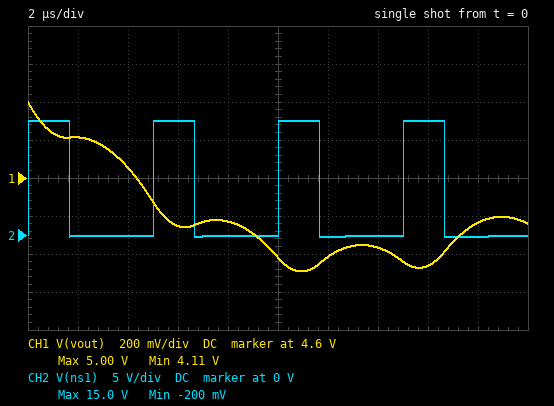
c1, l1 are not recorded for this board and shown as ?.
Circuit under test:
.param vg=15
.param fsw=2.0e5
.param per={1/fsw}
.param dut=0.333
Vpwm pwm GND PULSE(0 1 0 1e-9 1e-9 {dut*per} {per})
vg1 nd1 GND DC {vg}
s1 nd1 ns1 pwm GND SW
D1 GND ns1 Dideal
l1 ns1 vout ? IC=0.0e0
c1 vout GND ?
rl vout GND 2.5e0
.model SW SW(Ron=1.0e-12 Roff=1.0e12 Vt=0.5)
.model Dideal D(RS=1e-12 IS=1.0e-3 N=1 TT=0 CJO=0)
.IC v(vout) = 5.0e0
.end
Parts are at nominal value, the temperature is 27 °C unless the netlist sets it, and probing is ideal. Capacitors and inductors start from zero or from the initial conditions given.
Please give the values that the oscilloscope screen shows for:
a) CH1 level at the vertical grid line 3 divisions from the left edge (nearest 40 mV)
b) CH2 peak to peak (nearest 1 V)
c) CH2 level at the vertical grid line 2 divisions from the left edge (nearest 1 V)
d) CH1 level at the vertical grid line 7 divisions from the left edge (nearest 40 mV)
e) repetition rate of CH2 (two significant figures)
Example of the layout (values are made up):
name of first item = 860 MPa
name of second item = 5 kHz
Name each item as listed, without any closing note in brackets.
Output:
CH1 level at the vertical grid line 3 divisions from the left edge = 4.36 V
CH2 peak to peak = 15 V
CH2 level at the vertical grid line 2 divisions from the left edge = 0 V
CH1 level at the vertical grid line 7 divisions from the left edge = 4.24 V
repetition rate of CH2 = 200 kHz
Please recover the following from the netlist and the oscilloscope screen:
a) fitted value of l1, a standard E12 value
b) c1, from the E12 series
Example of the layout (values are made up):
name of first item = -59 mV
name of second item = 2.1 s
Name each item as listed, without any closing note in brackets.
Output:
fitted value of l1, a standard E12 value = 8.2 µH
c1, from the E12 series = 8.2 µF
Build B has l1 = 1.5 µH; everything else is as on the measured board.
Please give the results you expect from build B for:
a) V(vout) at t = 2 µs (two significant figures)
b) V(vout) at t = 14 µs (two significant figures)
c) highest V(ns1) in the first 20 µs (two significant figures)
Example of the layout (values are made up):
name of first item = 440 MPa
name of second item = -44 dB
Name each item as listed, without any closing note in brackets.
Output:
V(vout) at t = 2 µs = 6.0 V
V(vout) at t = 14 µs = 7.3 V
highest V(ns1) in the first 20 µs = 15 V
